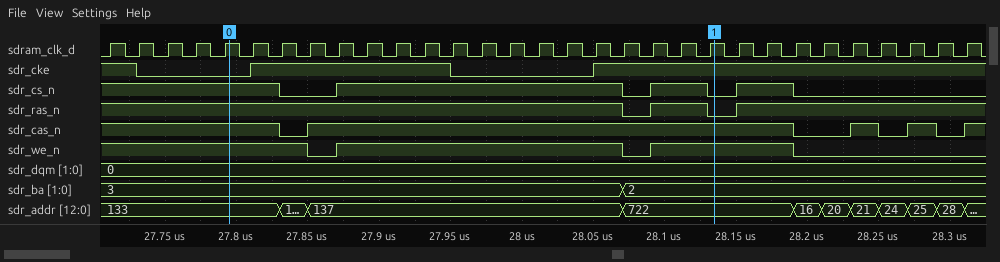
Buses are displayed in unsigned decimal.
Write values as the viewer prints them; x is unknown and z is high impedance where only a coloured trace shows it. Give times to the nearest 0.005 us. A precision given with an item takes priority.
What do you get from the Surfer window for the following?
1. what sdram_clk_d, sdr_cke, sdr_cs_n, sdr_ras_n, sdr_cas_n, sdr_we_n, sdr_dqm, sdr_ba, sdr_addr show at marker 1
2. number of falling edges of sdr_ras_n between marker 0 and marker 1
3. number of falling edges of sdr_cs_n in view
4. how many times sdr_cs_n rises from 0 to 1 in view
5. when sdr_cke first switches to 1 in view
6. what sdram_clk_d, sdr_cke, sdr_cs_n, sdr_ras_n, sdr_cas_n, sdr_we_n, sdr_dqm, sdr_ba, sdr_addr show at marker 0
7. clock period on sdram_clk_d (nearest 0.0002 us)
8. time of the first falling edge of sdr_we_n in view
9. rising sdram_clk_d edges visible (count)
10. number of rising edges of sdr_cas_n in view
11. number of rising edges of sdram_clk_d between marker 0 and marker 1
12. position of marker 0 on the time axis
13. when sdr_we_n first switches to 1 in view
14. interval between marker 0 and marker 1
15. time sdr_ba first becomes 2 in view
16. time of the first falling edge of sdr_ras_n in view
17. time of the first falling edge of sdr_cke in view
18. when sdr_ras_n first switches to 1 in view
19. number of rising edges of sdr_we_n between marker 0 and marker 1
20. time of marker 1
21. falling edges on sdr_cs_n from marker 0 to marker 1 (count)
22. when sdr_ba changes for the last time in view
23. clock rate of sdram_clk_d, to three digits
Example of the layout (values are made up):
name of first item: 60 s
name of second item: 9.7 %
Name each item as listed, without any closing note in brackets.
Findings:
what sdram_clk_d, sdr_cke, sdr_cs_n, sdr_ras_n, sdr_cas_n, sdr_we_n, sdr_dqm, sdr_ba, sdr_addr show at marker 1: sdram_clk_d=1, sdr_cke=1, sdr_cs_n=0, sdr_ras_n=0, sdr_cas_n=1, sdr_we_n=1, sdr_dqm=0, sdr_ba=2, sdr_addr=722
number of falling edges of sdr_ras_n between marker 0 and marker 1: 2
number of falling edges of sdr_cs_n in view: 4
how many times sdr_cs_n rises from 0 to 1 in view: 3
when sdr_cke first switches to 1 in view: 27.81 us
what sdram_clk_d, sdr_cke, sdr_cs_n, sdr_ras_n, sdr_cas_n, sdr_we_n, sdr_dqm, sdr_ba, sdr_addr show at marker 0: sdram_clk_d=1, sdr_cke=0, sdr_cs_n=1, sdr_ras_n=1, sdr_cas_n=1, sdr_we_n=1, sdr_dqm=0, sdr_ba=3, sdr_addr=133
clock period on sdram_clk_d: 0.02 us
time of the first falling edge of sdr_we_n in view: 27.85 us
rising sdram_clk_d edges visible: 31
number of rising edges of sdr_cas_n in view: 4
number of rising edges of sdram_clk_d between marker 0 and marker 1: 17
position of marker 0 on the time axis: 27.795 us
when sdr_we_n first switches to 1 in view: 27.87 us
interval between marker 0 and marker 1: 0.34 us
time sdr_ba first becomes 2 in view: 28.07 us
time of the first falling edge of sdr_ras_n in view: 28.07 us
time of the first falling edge of sdr_cke in view: 27.73 us
when sdr_ras_n first switches to 1 in view: 28.09 us
number of rising edges of sdr_we_n between marker 0 and marker 1: 2
time of marker 1: 28.135 us
falling edges on sdr_cs_n from marker 0 to marker 1: 3
when sdr_ba changes for the last time in view: 28.07 us
clock rate of sdram_clk_d, to three digits: 50.0 MHz
